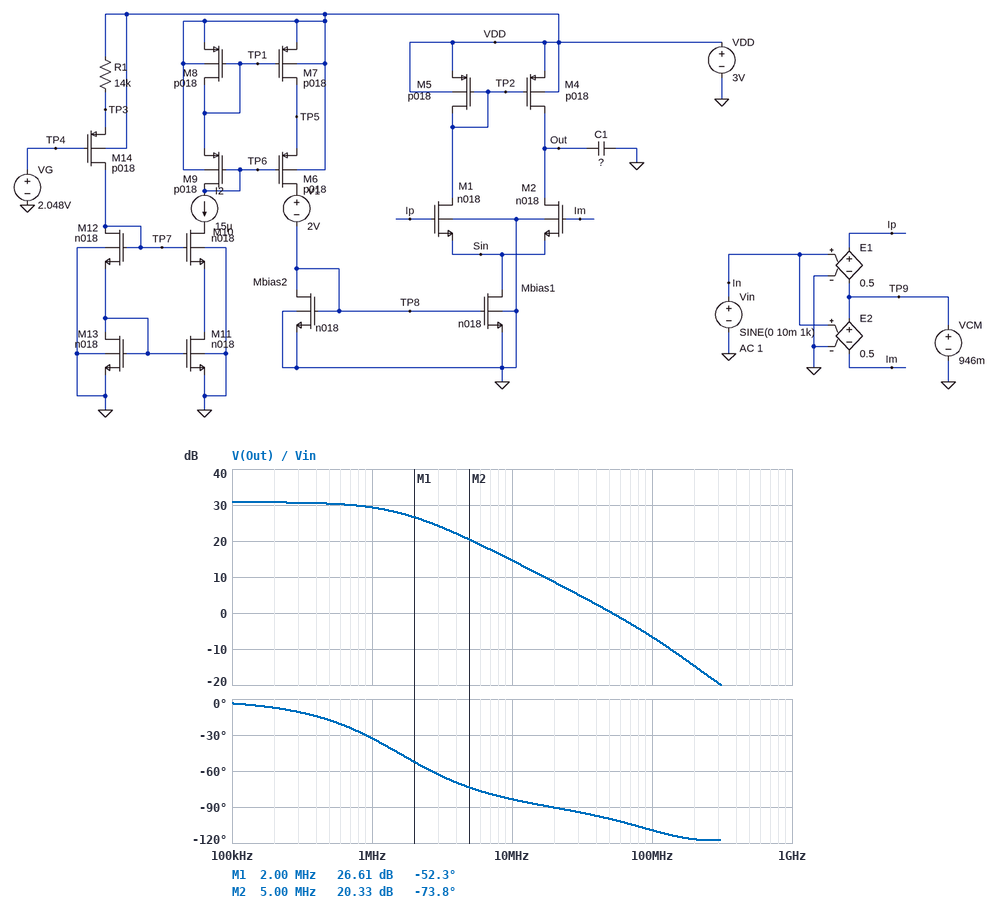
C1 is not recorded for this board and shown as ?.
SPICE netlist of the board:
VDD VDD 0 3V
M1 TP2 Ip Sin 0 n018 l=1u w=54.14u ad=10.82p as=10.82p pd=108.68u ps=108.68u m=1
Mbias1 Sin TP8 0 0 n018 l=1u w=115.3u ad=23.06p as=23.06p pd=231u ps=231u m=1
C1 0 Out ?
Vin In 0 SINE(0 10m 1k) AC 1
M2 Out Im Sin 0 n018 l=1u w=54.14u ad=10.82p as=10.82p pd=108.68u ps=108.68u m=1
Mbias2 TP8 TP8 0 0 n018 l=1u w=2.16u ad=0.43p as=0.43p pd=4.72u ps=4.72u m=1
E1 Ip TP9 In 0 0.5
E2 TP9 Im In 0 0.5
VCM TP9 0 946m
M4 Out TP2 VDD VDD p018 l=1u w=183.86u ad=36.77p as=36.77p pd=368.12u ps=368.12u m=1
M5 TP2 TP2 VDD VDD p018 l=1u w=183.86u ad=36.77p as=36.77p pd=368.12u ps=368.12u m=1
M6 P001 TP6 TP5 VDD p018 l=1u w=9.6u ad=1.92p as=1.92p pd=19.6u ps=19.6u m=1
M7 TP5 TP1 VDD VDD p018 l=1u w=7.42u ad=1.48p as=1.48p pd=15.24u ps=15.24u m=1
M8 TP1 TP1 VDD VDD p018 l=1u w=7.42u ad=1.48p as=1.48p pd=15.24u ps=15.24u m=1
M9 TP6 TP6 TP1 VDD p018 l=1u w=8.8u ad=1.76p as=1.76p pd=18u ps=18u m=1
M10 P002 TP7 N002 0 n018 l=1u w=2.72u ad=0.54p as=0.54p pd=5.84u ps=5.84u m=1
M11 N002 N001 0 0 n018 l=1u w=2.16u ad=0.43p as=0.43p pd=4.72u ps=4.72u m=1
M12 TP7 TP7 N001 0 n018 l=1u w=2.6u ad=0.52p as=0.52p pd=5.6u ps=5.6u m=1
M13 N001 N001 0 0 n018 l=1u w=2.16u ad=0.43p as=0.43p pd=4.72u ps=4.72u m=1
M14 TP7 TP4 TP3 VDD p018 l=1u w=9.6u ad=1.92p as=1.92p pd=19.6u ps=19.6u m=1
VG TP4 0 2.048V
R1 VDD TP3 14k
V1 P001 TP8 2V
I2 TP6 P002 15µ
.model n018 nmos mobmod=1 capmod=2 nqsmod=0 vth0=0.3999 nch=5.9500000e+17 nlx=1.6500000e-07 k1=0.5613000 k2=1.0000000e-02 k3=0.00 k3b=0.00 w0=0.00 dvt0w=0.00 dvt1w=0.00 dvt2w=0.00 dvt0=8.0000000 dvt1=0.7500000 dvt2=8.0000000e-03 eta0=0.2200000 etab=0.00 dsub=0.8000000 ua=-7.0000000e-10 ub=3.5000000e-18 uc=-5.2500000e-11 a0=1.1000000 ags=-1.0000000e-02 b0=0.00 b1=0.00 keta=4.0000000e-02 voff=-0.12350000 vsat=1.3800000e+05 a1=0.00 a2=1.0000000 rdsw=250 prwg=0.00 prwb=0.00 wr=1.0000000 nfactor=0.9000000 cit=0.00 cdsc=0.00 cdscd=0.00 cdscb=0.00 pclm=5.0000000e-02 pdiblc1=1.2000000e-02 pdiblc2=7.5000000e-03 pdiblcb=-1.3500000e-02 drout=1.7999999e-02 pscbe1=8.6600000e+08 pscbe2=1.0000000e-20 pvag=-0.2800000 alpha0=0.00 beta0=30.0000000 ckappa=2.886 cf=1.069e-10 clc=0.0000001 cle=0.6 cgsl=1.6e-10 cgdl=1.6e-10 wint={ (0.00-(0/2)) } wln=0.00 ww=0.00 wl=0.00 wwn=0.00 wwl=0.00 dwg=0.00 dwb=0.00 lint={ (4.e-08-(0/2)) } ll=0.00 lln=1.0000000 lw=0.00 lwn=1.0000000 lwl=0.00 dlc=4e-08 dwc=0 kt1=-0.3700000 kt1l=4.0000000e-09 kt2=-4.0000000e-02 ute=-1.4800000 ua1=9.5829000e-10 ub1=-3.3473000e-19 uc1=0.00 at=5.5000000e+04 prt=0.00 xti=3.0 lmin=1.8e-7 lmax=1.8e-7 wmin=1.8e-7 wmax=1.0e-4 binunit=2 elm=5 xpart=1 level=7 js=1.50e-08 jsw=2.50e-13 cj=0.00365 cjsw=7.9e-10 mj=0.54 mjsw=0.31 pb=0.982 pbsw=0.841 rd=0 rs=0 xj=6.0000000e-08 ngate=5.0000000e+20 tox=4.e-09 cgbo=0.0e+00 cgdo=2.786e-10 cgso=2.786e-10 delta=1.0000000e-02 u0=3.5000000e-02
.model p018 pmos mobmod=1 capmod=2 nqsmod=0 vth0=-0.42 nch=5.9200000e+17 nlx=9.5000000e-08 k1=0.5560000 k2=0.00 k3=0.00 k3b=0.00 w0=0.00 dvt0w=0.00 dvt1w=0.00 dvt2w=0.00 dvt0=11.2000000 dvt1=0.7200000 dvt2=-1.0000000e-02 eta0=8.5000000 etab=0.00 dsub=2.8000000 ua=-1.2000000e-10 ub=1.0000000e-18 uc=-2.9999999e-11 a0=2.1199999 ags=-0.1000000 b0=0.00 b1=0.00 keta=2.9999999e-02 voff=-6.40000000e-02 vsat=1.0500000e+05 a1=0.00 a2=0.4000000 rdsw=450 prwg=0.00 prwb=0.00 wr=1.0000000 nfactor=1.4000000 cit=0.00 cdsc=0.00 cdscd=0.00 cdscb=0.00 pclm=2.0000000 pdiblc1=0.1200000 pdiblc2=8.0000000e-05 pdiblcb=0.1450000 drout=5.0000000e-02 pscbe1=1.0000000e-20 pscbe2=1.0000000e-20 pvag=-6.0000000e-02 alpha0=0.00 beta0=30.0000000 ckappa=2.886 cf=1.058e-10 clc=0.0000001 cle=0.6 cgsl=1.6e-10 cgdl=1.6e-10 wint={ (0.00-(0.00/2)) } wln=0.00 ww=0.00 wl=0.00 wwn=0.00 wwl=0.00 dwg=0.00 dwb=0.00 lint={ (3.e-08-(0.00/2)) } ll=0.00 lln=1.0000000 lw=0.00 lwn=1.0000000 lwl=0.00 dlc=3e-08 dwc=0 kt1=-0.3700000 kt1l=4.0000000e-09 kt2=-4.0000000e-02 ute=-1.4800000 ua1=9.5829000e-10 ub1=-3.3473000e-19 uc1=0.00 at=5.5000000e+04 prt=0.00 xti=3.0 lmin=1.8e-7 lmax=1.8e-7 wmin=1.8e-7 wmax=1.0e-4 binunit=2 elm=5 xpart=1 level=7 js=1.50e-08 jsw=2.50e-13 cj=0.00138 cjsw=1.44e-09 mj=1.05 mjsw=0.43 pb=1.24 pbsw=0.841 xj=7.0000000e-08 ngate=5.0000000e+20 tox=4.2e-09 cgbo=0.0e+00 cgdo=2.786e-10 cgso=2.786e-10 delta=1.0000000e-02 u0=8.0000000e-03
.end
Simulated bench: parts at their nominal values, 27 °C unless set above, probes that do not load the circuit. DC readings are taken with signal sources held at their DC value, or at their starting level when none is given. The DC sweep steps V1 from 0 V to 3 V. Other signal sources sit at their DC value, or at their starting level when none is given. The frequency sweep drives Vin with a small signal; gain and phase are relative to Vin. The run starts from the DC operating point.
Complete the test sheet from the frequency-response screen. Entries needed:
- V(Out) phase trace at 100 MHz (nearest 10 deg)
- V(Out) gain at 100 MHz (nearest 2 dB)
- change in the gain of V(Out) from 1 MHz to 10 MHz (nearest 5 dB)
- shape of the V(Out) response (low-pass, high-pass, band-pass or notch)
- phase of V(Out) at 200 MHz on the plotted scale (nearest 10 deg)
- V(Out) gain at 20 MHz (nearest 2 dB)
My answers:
-110 deg
-6 dB
-15 dB
low-pass
-120 deg
8 dB
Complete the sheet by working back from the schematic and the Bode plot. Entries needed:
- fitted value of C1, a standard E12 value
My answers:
6.8 pF
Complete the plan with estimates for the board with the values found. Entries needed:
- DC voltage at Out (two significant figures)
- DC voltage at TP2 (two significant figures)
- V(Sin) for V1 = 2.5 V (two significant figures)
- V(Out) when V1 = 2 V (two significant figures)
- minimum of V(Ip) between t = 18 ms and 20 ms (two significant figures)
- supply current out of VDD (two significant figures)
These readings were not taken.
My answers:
2.2 V
2.2 V
400 mV
2.2 V
940 mV
1.0 mA
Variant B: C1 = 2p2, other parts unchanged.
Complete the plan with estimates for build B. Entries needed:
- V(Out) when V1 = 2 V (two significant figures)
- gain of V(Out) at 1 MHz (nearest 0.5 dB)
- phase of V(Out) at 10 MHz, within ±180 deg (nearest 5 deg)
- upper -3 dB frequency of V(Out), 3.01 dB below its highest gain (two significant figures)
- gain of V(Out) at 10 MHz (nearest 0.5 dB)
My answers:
2.2 V
30.5 dB
-70 deg
4.1 MHz
22.5 dB
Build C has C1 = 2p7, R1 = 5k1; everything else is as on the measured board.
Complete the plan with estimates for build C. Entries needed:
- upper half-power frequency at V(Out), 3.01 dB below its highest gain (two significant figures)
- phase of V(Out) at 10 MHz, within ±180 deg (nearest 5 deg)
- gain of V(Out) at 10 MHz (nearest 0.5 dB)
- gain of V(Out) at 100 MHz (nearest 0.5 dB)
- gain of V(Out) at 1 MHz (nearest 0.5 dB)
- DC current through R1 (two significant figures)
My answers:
3.5 MHz
-75 deg
21.0 dB
0.5 dB
30.5 dB
26 µA
